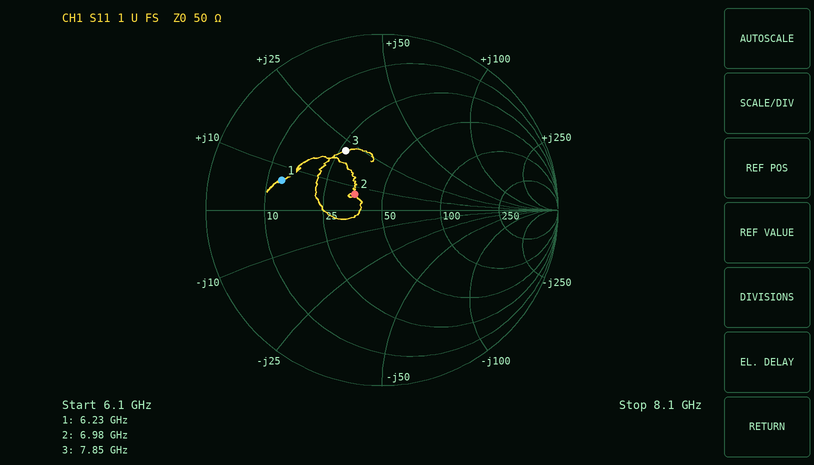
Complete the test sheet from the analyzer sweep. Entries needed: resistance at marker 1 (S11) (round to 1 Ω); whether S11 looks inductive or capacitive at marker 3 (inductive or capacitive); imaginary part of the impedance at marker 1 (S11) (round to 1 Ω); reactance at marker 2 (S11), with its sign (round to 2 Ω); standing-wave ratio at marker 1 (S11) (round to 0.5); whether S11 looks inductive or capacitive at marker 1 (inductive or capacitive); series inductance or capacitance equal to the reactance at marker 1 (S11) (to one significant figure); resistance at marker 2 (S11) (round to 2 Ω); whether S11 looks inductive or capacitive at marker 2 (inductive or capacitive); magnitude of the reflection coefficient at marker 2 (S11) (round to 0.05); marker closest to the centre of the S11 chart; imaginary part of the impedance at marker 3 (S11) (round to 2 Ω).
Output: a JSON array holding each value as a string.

["13 Ω", "inductive", "+7 Ω", "+6 Ω", "4.0", "inductive", "200 pH", "36 Ω", "inductive", "0.20", "marker 2", "+22 Ω"]
